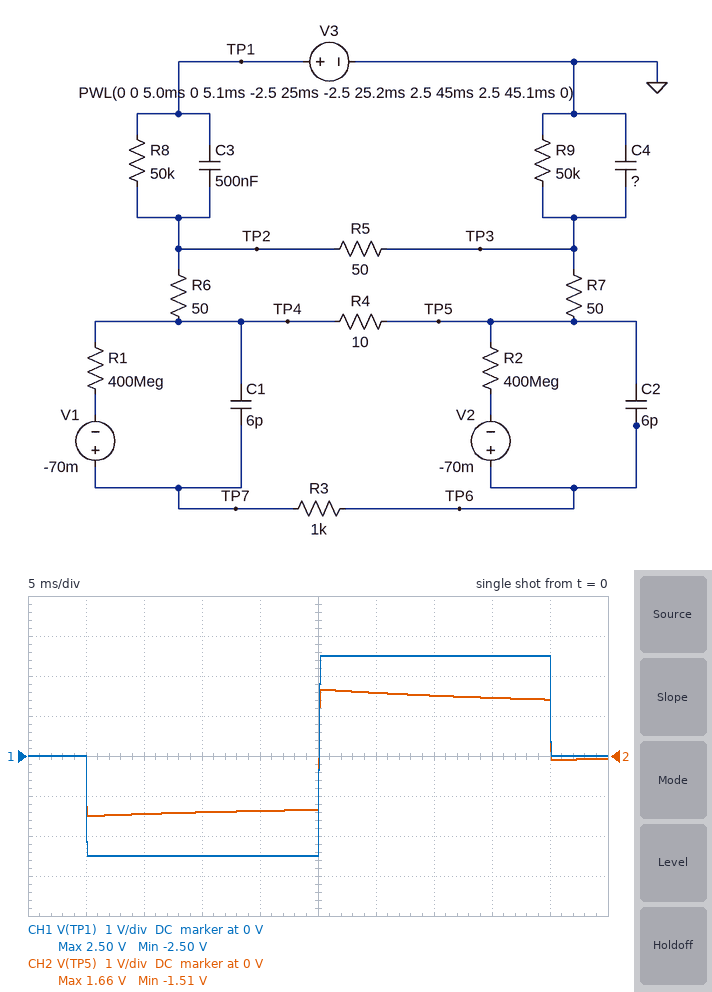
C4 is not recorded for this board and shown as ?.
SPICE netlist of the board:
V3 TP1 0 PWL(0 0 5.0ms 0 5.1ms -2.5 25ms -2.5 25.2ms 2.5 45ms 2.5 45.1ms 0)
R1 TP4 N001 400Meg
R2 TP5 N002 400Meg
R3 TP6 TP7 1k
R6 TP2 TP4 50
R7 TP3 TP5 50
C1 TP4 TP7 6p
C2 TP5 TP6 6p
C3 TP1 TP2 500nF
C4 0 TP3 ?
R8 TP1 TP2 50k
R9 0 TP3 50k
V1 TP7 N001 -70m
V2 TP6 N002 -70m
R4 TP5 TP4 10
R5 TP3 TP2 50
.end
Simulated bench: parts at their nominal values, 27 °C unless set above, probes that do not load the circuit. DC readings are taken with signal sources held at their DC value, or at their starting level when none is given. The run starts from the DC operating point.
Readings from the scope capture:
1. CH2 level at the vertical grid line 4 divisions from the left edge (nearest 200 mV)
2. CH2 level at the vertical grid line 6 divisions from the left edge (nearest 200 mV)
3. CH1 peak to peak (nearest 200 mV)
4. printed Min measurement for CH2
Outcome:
-1.4 V
1.6 V
5.0 V
-1.51 V
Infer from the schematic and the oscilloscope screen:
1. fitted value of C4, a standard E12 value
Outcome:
330 nF
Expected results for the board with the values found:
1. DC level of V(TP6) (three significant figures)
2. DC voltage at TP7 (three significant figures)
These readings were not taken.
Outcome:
-70.0 mV
-70.0 mV
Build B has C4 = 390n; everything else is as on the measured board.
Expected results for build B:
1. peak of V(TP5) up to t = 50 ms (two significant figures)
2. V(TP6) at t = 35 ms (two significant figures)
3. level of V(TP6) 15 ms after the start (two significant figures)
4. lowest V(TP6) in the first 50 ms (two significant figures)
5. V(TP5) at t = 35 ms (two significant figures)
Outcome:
1.5 V
1.3 V
-1.4 V
-1.5 V
1.4 V
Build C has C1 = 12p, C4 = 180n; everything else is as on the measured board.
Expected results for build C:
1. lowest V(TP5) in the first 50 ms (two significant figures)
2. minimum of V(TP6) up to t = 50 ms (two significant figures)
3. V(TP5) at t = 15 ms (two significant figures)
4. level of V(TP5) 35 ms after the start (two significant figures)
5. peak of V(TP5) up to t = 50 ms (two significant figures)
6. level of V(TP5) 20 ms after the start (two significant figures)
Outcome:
-1.8 V
-1.9 V
-1.6 V
1.8 V
2.2 V
-1.5 V
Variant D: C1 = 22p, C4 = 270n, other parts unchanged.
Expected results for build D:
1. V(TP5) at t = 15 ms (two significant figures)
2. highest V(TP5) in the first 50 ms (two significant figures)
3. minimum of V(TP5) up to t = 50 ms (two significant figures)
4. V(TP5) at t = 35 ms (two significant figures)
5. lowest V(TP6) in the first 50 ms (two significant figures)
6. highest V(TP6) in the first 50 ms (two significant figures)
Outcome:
-1.5 V
1.9 V
-1.6 V
1.6 V
-1.7 V
1.8 V
